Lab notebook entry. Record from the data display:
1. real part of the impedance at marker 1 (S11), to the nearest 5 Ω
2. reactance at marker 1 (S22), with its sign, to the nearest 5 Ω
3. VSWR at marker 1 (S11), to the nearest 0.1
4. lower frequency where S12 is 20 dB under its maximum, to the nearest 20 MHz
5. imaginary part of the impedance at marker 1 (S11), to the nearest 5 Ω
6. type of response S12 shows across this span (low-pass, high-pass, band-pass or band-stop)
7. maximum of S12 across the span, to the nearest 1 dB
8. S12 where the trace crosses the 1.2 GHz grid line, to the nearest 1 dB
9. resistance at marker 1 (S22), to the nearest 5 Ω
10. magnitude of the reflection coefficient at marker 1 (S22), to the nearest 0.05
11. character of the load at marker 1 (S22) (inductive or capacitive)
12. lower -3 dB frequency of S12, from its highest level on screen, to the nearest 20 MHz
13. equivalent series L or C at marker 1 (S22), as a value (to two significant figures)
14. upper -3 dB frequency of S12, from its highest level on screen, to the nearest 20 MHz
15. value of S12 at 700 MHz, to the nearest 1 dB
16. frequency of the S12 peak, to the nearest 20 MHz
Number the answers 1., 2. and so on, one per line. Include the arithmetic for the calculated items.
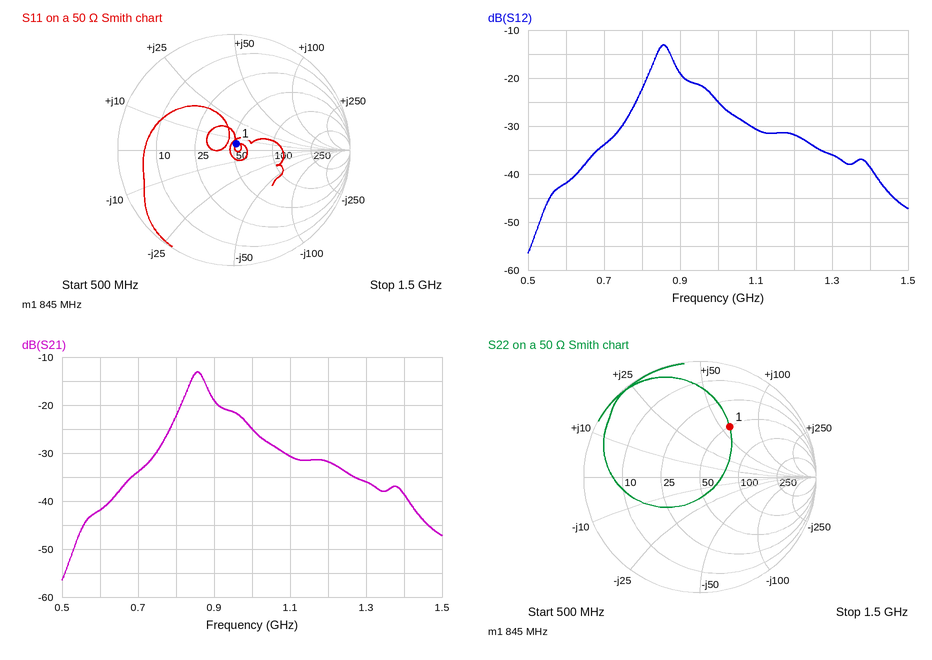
1. 50 Ω
2. +60 Ω
3. 1.1
4. 720 MHz
5. +5 Ω
6. band-pass
7. -13 dB
8. -32 dB
9. 50 Ω
10. 0.50
11. inductive
12. 840 MHz
13. L = 60 Ω/(2π × 845 MHz) ≈ 11 nH
14. 880 MHz
15. -34 dB
16. 860 MHz
